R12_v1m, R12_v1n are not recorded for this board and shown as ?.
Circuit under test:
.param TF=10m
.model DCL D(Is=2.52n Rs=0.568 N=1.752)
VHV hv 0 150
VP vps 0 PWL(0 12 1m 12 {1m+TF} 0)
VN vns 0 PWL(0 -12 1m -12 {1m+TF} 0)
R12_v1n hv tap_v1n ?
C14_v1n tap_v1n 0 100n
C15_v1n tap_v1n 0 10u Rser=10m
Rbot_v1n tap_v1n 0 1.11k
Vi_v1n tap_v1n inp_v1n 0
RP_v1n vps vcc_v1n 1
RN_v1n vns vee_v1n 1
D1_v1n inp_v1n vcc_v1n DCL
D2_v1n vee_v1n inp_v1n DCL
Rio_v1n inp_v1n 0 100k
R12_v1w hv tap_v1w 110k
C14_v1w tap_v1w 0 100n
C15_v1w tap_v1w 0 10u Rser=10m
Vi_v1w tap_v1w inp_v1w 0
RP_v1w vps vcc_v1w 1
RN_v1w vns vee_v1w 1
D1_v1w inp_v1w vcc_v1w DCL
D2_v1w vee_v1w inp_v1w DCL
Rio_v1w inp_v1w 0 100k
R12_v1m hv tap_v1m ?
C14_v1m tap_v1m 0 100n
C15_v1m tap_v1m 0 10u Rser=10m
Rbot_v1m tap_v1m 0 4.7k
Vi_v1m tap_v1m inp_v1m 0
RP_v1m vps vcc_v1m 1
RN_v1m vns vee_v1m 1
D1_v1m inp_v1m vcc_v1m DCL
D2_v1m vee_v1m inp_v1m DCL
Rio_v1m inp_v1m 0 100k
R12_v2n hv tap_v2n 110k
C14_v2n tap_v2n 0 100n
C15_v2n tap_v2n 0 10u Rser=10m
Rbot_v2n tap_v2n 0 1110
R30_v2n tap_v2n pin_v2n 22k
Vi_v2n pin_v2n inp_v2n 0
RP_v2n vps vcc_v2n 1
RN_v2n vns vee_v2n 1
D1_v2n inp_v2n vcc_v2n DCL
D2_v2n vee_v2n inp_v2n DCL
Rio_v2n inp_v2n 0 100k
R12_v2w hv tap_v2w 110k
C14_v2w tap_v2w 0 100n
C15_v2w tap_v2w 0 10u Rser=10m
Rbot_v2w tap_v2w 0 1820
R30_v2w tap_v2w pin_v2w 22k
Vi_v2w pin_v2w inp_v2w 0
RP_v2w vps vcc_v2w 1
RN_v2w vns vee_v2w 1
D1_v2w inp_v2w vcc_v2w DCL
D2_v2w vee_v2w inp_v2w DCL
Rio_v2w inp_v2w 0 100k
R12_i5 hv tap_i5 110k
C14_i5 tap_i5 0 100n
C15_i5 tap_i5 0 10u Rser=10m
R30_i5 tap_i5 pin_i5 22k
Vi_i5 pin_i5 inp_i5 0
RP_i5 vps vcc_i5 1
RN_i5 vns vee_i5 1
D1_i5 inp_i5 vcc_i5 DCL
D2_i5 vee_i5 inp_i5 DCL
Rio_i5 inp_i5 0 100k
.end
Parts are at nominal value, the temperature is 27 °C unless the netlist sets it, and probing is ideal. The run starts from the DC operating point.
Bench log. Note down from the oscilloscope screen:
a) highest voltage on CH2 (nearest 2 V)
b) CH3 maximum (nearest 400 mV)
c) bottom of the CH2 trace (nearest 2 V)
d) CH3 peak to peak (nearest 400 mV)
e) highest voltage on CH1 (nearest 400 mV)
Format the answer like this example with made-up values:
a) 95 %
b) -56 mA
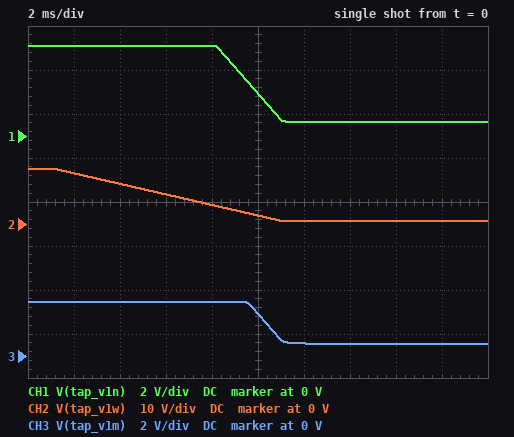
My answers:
a) 12 V
b) 2.4 V
c) 0 V
d) 2.0 V
e) 4.0 V
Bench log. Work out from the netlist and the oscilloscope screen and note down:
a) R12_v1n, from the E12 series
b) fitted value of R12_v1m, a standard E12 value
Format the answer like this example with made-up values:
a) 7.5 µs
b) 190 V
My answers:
a) 39 kΩ
b) 270 kΩ
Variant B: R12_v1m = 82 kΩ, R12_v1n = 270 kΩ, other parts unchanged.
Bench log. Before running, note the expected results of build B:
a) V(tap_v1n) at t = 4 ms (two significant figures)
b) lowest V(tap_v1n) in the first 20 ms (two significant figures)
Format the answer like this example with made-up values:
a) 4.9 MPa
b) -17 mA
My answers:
a) 610 mV
b) 490 mV
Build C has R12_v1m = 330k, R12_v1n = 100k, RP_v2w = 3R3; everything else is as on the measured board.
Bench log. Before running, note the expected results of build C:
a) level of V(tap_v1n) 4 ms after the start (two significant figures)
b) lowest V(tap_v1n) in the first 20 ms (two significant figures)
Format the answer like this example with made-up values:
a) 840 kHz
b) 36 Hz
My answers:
a) 1.6 V
b) 580 mV
